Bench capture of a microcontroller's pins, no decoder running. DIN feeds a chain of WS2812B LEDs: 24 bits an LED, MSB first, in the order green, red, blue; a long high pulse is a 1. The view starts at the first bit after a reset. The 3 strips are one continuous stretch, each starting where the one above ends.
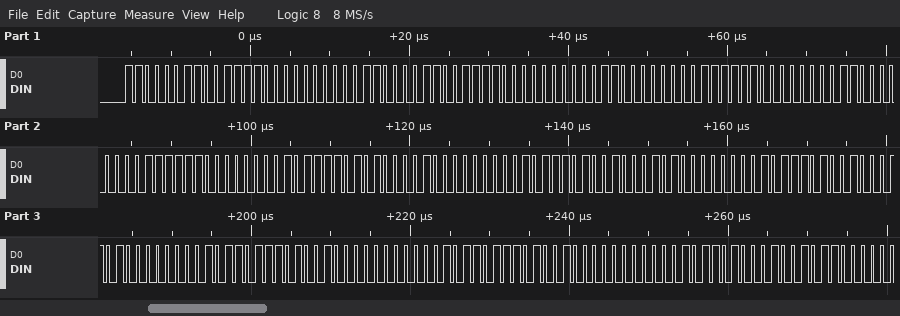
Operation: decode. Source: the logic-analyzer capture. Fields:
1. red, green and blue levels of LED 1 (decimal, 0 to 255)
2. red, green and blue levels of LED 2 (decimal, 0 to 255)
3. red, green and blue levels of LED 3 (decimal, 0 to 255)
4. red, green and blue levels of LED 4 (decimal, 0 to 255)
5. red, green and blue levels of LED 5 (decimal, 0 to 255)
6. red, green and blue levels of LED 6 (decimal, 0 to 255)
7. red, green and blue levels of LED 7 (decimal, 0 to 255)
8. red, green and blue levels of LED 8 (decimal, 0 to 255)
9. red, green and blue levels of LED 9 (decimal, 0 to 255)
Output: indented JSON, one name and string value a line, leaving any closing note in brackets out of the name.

{
  "red, green and blue levels of LED 1": "60, 195, 0",
  "red, green and blue levels of LED 2": "60, 195, 0",
  "red, green and blue levels of LED 3": "63, 192, 0",
  "red, green and blue levels of LED 4": "63, 192, 0",
  "red, green and blue levels of LED 5": "66, 189, 0",
  "red, green and blue levels of LED 6": "69, 186, 0",
  "red, green and blue levels of LED 7": "69, 186, 0",
  "red, green and blue levels of LED 8": "72, 183, 0",
  "red, green and blue levels of LED 9": "72, 183, 0"
}
